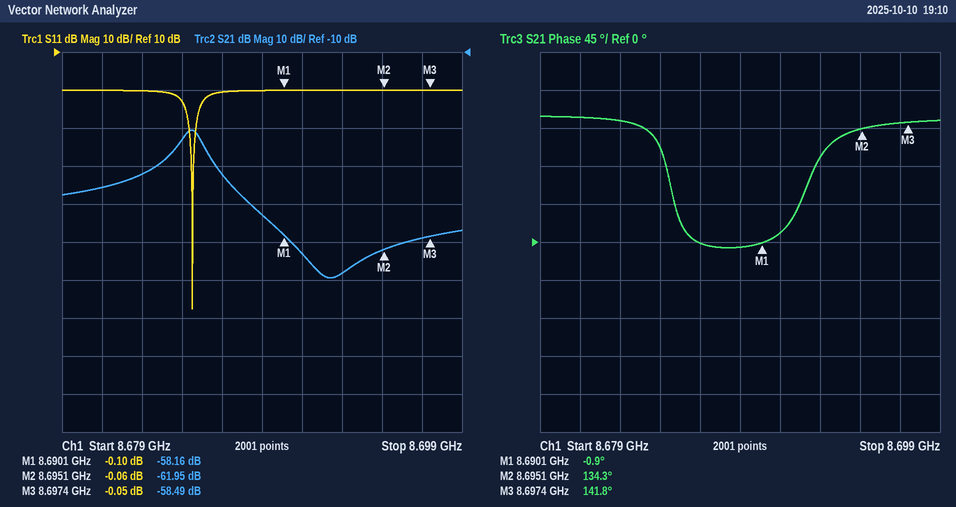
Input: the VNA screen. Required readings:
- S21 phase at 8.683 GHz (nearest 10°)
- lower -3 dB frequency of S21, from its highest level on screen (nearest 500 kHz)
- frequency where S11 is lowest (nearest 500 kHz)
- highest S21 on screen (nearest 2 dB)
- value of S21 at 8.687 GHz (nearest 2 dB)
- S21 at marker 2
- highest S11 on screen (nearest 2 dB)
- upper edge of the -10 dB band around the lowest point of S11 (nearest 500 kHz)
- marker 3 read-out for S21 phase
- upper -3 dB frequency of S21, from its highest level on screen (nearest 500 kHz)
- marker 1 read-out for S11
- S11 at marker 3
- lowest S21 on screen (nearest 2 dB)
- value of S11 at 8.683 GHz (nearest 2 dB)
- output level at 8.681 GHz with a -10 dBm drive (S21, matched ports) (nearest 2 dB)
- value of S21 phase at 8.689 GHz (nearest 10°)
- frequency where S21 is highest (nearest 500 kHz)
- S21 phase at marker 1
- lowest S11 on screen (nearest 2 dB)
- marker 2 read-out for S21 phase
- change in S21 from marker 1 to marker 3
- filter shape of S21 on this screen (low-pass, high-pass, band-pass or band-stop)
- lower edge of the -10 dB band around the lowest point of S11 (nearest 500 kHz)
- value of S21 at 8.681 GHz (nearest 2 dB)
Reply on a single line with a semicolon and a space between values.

140°; 8.6850 GHz; 8.6855 GHz; -30 dB; -42 dB; -61.95 dB; 0 dB; 8.6855 GHz; 141.8°; 8.6860 GHz; -0.10 dB; -0.05 dB; -70 dB; 0 dB; -56 dBm; -10°; 8.6855 GHz; -0.9°; -58 dB; 134.3°; -0.33 dB; band-pass; 8.6855 GHz; -46 dB
